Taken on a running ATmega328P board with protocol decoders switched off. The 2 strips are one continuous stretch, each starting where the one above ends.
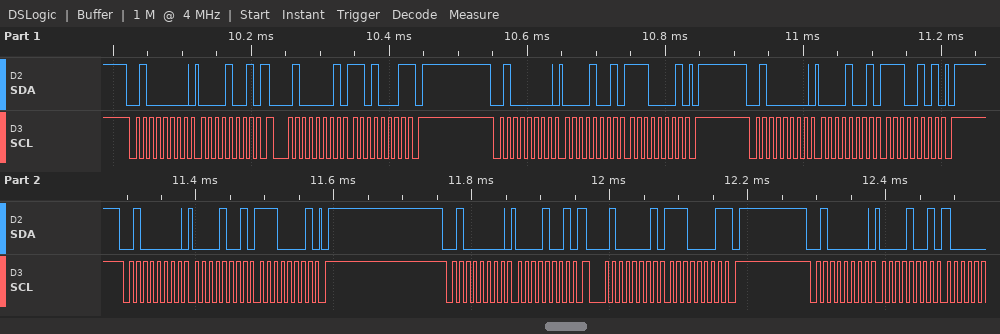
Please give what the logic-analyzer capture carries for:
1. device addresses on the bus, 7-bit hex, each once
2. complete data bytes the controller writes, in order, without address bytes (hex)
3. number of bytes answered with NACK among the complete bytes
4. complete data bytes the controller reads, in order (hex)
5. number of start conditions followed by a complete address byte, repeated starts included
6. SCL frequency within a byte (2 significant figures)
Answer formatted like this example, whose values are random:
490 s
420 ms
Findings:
0x20
09 09 E1 09 E5 09 E1 09 09
2
D1 E1
8
100 kHz
